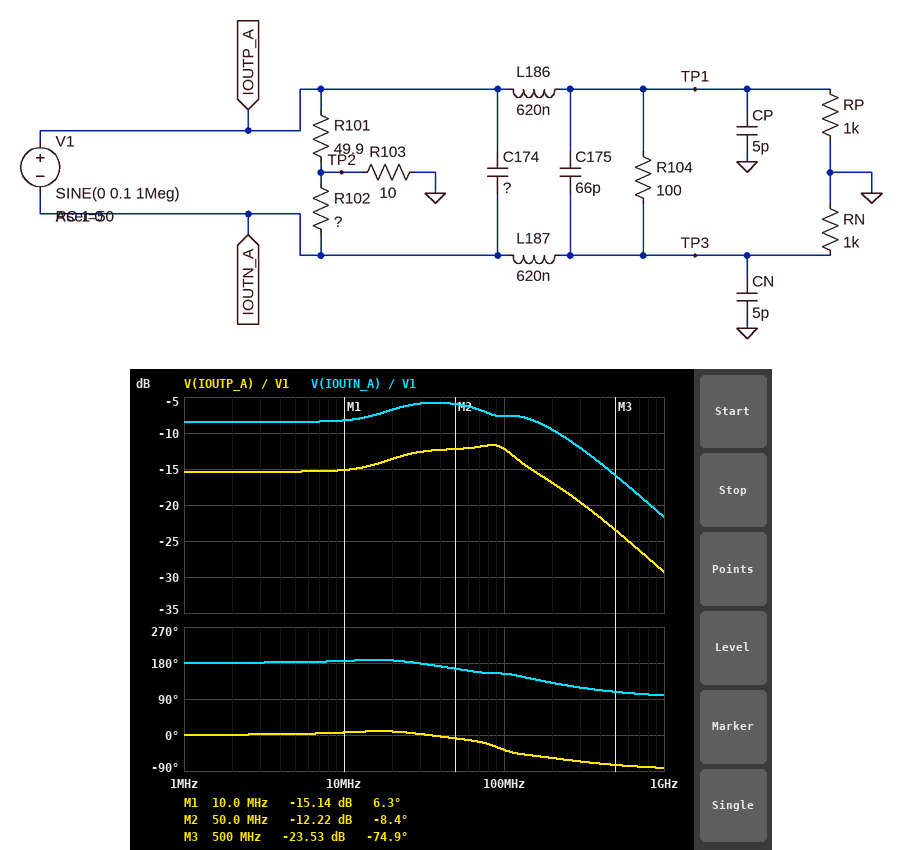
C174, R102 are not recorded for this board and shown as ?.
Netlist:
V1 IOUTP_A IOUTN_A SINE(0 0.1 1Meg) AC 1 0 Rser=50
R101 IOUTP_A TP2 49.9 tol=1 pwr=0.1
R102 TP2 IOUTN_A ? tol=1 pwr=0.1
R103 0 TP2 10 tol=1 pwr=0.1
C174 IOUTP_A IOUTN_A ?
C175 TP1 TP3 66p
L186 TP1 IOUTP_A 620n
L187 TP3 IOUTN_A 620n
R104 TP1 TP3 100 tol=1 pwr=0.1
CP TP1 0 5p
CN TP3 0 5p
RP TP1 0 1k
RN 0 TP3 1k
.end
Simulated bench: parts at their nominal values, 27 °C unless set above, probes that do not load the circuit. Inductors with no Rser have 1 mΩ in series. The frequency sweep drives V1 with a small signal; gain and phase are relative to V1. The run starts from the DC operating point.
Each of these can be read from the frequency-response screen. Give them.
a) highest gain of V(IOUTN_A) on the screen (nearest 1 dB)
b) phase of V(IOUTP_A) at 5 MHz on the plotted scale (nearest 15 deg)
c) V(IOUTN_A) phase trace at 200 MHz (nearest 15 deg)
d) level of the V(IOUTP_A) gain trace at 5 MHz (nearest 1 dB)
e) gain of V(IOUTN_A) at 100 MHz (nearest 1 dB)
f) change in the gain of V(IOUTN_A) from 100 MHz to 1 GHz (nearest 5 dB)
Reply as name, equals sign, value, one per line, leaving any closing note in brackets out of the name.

highest gain of V(IOUTN_A) on the screen = -6 dB
phase of V(IOUTP_A) at 5 MHz on the plotted scale = 0 deg
V(IOUTN_A) phase trace at 200 MHz = 135 deg
level of the V(IOUTP_A) gain trace at 5 MHz = -15 dB
gain of V(IOUTN_A) at 100 MHz = -8 dB
change in the gain of V(IOUTN_A) from 100 MHz to 1 GHz = -15 dB
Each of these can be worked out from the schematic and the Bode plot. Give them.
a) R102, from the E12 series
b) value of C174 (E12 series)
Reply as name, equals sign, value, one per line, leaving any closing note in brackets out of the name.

R102, from the E12 series = 120 Ω
value of C174 = 27 pF
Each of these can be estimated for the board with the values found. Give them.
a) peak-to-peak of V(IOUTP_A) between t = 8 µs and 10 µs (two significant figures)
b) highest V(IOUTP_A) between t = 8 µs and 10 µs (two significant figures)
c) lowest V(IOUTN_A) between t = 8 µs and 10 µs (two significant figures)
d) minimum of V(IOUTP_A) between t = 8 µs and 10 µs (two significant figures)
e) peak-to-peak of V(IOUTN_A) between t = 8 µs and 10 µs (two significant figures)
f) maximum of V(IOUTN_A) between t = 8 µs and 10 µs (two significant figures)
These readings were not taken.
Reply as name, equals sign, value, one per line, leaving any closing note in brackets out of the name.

peak-to-peak of V(IOUTP_A) between t = 8 µs and 10 µs = 34 mV
highest V(IOUTP_A) between t = 8 µs and 10 µs = 17 mV
lowest V(IOUTN_A) between t = 8 µs and 10 µs = -38 mV
minimum of V(IOUTP_A) between t = 8 µs and 10 µs = -17 mV
peak-to-peak of V(IOUTN_A) between t = 8 µs and 10 µs = 76 mV
maximum of V(IOUTN_A) between t = 8 µs and 10 µs = 38 mV
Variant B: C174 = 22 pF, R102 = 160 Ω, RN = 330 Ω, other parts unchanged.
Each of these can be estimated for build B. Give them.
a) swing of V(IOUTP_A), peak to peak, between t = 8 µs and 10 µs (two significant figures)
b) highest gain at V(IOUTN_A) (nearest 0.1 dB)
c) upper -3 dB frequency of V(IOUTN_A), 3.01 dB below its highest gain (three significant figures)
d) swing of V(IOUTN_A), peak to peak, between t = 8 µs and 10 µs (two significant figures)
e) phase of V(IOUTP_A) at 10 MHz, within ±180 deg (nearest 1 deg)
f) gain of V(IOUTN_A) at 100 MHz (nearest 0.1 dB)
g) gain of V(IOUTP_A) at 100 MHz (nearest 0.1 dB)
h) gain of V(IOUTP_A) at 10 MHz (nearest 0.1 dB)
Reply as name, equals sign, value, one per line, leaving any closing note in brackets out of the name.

swing of V(IOUTP_A), peak to peak, between t = 8 µs and 10 µs = 35 mV
highest gain at V(IOUTN_A) = -5.0 dB
upper -3 dB frequency of V(IOUTN_A), 3.01 dB below its highest gain = 213 MHz
swing of V(IOUTN_A), peak to peak, between t = 8 µs and 10 µs = 75 mV
phase of V(IOUTP_A) at 10 MHz, within ±180 deg = 2 deg
gain of V(IOUTN_A) at 100 MHz = -6.1 dB
gain of V(IOUTP_A) at 100 MHz = -13.0 dB
gain of V(IOUTP_A) at 10 MHz = -15.2 dB
